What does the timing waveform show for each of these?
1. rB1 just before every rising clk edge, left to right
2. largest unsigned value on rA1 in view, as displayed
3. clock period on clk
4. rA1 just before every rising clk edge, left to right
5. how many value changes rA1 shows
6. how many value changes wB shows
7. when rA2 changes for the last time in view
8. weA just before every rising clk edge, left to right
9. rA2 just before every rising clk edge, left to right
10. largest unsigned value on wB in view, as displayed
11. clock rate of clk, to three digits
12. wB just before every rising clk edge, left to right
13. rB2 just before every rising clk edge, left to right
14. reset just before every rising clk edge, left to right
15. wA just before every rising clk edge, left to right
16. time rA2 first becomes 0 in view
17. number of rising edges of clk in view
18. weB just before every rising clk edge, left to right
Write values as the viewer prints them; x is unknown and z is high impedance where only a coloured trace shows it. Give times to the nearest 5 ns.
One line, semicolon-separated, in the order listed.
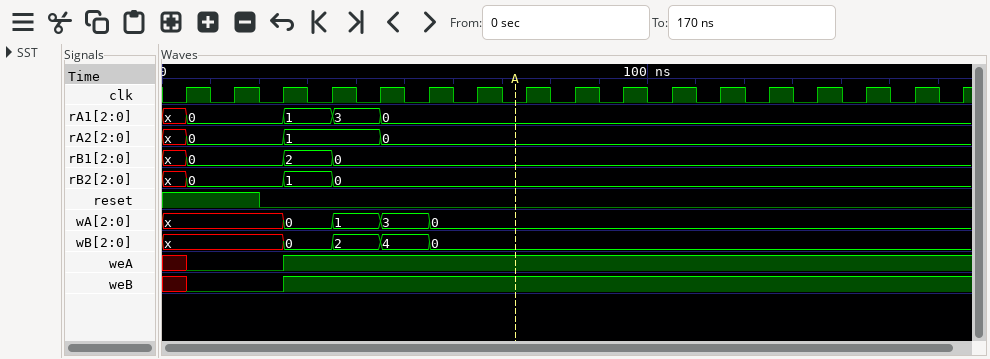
x, 0, 0, 2, 0, 0, 0, 0, 0, 0, 0, 0, 0, 0, 0, 0, 0; 3; 10 ns; x, 0, 0, 1, 3, 0, 0, 0, 0, 0, 0, 0, 0, 0, 0, 0, 0; 4; 4; 45 ns; x 0 0 1 1 1 1 1 1 1 1 1 1 1 1 1 1; x, 0, 0, 1, 1, 0, 0, 0, 0, 0, 0, 0, 0, 0, 0, 0, 0; 4; 100 MHz; x, x, x, 0, 2, 4, 0, 0, 0, 0, 0, 0, 0, 0, 0, 0, 0; x, 0, 0, 1, 0, 0, 0, 0, 0, 0, 0, 0, 0, 0, 0, 0, 0; 1 1 0 0 0 0 0 0 0 0 0 0 0 0 0 0 0; x, x, x, 0, 1, 3, 0, 0, 0, 0, 0, 0, 0, 0, 0, 0, 0; 5 ns; 17; x 0 0 1 1 1 1 1 1 1 1 1 1 1 1 1 1
